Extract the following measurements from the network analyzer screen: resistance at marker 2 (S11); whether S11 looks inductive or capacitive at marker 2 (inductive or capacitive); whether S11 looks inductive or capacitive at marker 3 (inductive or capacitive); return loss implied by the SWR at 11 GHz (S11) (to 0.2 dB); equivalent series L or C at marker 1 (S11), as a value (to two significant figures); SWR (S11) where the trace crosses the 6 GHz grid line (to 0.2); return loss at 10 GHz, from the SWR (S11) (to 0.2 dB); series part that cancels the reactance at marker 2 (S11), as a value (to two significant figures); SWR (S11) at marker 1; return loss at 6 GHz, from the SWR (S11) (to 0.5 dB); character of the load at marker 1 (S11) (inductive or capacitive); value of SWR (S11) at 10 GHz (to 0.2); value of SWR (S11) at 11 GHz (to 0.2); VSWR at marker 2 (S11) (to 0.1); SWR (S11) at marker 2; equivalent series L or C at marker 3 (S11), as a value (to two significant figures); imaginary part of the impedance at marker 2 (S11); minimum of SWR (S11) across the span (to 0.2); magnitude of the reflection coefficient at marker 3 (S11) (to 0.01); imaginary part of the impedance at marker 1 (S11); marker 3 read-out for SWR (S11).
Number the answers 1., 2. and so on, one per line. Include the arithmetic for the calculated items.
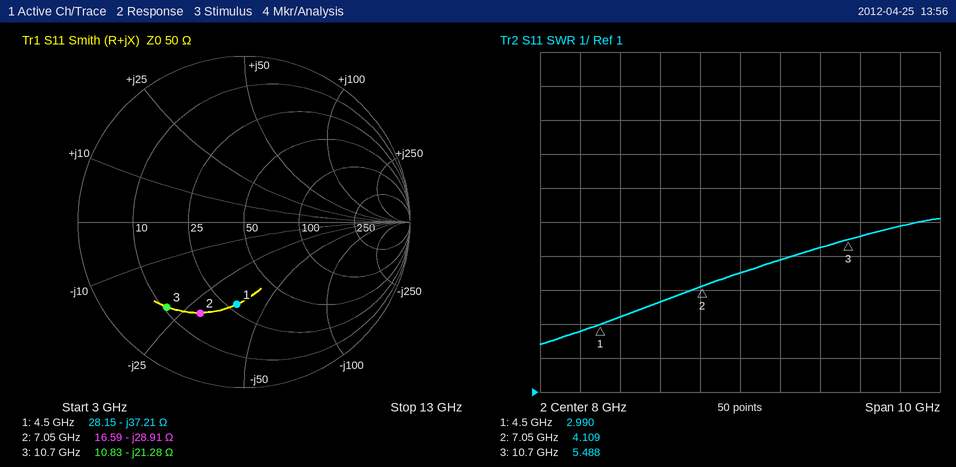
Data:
1. 16.59 Ω
2. capacitive
3. capacitive
4. −20 log10((5.6 − 1)/(5.6 + 1)) ≈ 3.14 dB, so 3.2 dB to the nearest 0.2 dB
5. C = 1/(2π × 4.5 GHz × 37.21 Ω) ≈ 950 fF
6. 3.6
7. −20 log10((5.2 − 1)/(5.2 + 1)) ≈ 3.4 dB
8. L = 28.91 Ω/(2π × 7.05 GHz) ≈ 653 pH, so 650 pH to two significant figures
9. 2.990
10. −20 log10((3.6 − 1)/(3.6 + 1)) ≈ 5.0 dB
11. capacitive
12. 5.2
13. 5.6
14. 4.1
15. 4.109
16. C = 1/(2π × 10.7 GHz × 21.28 Ω) ≈ 699 fF, so 700 fF to two significant figures
17. -28.91 Ω
18. 2.4
19. 0.69
20. -37.21 Ω
21. 5.488
